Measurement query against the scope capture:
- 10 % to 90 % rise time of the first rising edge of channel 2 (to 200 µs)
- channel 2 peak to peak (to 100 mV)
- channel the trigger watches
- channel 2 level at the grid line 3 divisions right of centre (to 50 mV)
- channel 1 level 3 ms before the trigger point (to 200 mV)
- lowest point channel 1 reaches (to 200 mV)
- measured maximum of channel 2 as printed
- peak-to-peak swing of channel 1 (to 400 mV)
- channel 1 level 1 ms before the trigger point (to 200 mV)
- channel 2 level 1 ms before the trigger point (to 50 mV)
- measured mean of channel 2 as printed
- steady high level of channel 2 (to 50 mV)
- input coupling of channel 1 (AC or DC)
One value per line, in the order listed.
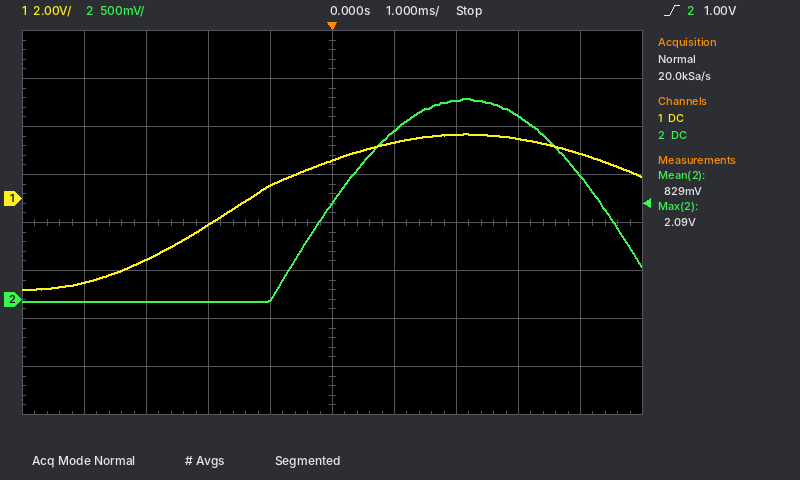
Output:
2.0 ms
2.10 V
channel 2
1.90 V
-2.6 V
-3.8 V
2.09 V
6.4 V
600 mV
0 mV
829 mV
2.05 V
DC
